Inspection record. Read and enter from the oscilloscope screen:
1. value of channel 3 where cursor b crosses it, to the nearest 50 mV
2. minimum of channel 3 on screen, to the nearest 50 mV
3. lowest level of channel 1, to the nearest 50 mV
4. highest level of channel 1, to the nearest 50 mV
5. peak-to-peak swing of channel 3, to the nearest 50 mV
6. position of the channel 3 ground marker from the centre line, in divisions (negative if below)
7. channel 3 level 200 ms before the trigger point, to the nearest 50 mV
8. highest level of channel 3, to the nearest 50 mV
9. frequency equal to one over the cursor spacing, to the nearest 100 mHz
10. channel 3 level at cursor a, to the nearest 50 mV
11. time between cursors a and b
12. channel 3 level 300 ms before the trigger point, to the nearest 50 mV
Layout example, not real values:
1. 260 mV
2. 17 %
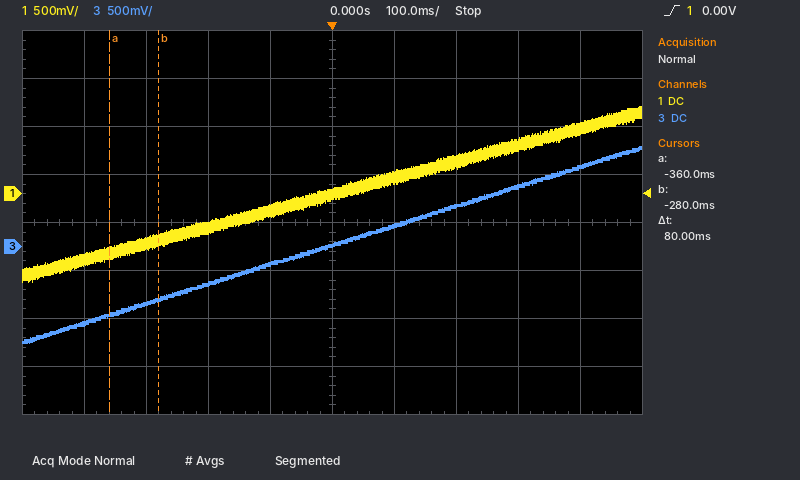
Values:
1. -550 mV
2. -1.00 V
3. -900 mV
4. 900 mV
5. 2.05 V
6. -0.5 div
7. -400 mV
8. 1.05 V
9. 12.5 Hz
10. -700 mV
11. 80 ms
12. -600 mV
